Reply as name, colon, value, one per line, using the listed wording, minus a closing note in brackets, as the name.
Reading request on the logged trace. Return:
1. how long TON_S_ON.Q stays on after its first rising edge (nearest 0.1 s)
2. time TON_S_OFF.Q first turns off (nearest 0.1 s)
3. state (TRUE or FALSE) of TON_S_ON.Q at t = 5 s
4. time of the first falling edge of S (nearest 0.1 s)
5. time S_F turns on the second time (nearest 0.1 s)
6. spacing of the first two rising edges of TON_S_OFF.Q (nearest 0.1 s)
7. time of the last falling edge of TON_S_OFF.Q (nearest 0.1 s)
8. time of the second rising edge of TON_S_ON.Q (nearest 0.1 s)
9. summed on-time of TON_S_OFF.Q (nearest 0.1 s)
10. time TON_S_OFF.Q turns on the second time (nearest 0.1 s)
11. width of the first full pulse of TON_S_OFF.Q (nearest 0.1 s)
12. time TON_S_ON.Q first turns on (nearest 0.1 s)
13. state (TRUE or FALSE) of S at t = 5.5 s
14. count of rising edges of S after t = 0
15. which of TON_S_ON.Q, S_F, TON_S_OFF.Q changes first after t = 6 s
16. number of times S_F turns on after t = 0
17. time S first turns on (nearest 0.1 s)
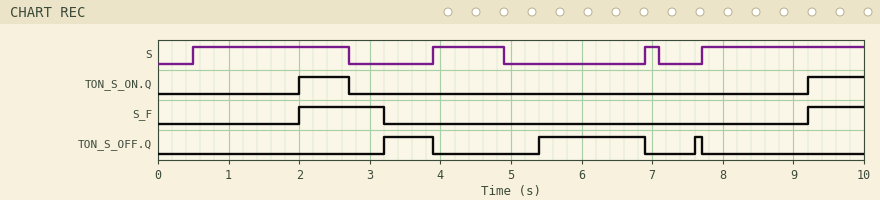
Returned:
how long TON_S_ON.Q stays on after its first rising edge: 0.7 s
time TON_S_OFF.Q first turns off: 3.9 s
state (TRUE or FALSE) of TON_S_ON.Q at t = 5 s: FALSE
time of the first falling edge of S: 2.7 s
time S_F turns on the second time: 9.2 s
spacing of the first two rising edges of TON_S_OFF.Q: 2.2 s
time of the last falling edge of TON_S_OFF.Q: 7.7 s
time of the second rising edge of TON_S_ON.Q: 9.2 s
summed on-time of TON_S_OFF.Q: 2.3 s
time TON_S_OFF.Q turns on the second time: 5.4 s
width of the first full pulse of TON_S_OFF.Q: 0.7 s
time TON_S_ON.Q first turns on: 2.0 s
state (TRUE or FALSE) of S at t = 5.5 s: FALSE
count of rising edges of S after t = 0: 4
which of TON_S_ON.Q, S_F, TON_S_OFF.Q changes first after t = 6 s: TON_S_OFF.Q
number of times S_F turns on after t = 0: 2
time S first turns on: 0.5 s
